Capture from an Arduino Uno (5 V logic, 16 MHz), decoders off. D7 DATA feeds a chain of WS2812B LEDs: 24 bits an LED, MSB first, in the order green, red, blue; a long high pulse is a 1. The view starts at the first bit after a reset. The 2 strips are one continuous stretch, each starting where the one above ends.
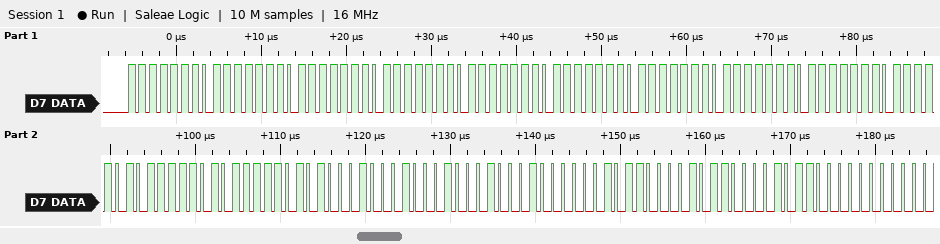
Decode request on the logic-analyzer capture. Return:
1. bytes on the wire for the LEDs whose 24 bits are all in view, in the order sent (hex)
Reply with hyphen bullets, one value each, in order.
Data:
- FE FE FE FE FE FE FE FE FE FA FA FA 88 88 88 16 16 16
